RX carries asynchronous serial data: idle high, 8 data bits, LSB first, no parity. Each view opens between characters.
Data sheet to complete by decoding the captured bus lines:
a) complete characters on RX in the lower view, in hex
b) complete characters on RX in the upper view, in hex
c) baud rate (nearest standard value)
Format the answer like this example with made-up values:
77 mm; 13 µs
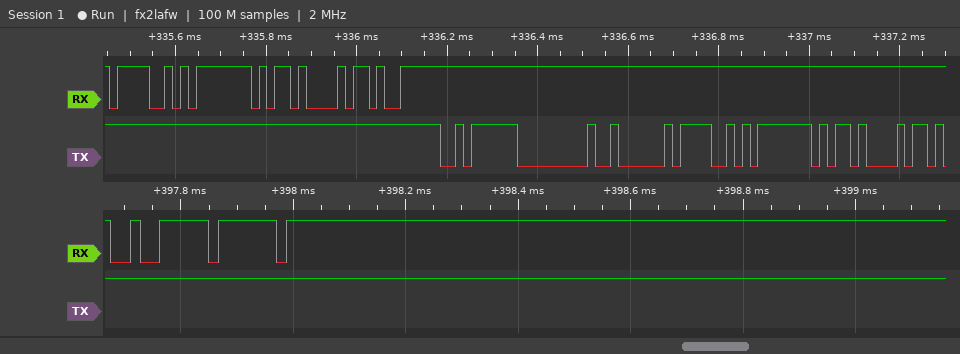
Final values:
F2, BF; 4F, 7F, 0B, CB; 57600 baud
